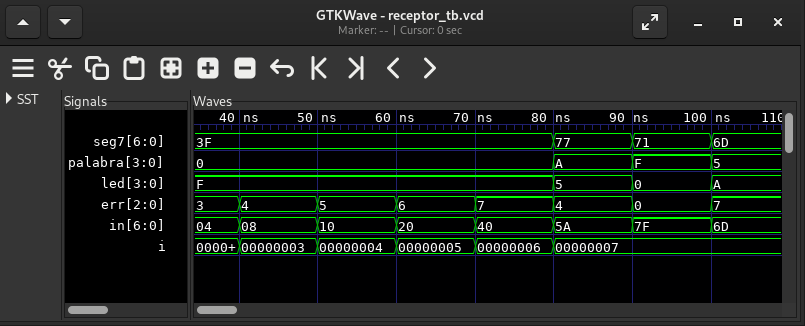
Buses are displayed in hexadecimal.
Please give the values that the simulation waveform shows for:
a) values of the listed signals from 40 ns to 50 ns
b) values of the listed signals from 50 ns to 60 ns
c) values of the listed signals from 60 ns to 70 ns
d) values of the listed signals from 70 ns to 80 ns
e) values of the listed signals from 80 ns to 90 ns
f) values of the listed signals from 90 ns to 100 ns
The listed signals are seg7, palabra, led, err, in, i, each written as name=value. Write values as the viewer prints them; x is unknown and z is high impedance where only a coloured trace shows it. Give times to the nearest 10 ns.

seg7=3F, palabra=0, led=F, err=4, in=08, i=00000003
seg7=3F, palabra=0, led=F, err=5, in=10, i=00000004
seg7=3F, palabra=0, led=F, err=6, in=20, i=00000005
seg7=3F, palabra=0, led=F, err=7, in=40, i=00000006
seg7=77, palabra=A, led=5, err=4, in=5A, i=00000007
seg7=71, palabra=F, led=0, err=0, in=7F, i=00000007
